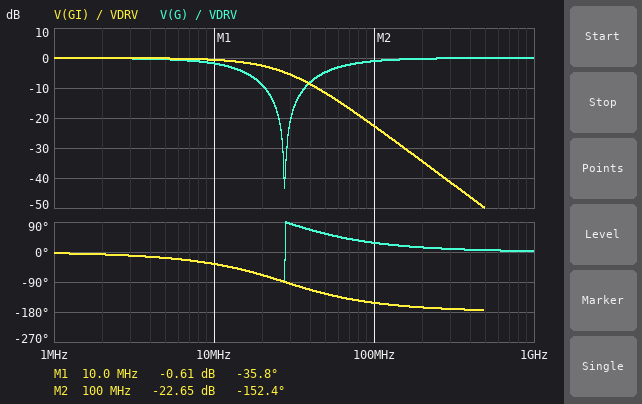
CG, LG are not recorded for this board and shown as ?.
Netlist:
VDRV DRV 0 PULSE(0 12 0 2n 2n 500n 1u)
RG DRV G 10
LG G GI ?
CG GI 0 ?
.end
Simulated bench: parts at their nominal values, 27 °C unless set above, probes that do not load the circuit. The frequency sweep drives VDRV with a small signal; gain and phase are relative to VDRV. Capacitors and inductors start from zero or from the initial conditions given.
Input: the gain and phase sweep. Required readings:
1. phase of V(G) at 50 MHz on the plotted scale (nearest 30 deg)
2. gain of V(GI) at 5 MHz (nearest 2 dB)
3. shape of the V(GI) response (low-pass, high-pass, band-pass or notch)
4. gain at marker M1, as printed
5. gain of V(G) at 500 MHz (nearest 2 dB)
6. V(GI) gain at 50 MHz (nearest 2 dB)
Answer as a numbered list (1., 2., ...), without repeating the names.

1. 60 deg
2. 0 dB
3. low-pass
4. -0.61 dB
5. 0 dB
6. -12 dB
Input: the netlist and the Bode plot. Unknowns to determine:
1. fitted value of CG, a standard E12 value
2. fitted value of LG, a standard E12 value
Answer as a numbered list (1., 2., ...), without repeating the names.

1. 1 nF
2. 33 nH
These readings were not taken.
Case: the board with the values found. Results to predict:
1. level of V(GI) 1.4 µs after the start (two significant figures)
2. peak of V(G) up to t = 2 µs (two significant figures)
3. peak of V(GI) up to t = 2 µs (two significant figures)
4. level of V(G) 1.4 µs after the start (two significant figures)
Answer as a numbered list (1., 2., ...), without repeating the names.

1. 12 V
2. 12 V
3. 12 V
4. 12 V
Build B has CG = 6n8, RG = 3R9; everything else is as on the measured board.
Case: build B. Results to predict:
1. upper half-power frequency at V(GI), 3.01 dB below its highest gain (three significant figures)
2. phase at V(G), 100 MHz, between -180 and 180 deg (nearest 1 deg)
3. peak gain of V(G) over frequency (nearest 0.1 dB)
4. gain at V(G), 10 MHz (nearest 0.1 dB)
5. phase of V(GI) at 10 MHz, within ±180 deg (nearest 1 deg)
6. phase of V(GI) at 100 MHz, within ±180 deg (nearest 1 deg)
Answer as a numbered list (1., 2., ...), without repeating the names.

1. 8.11 MHz
2. 11 deg
3. 0 dB
4. -23.3 dB
5. -86 deg
6. -169 deg
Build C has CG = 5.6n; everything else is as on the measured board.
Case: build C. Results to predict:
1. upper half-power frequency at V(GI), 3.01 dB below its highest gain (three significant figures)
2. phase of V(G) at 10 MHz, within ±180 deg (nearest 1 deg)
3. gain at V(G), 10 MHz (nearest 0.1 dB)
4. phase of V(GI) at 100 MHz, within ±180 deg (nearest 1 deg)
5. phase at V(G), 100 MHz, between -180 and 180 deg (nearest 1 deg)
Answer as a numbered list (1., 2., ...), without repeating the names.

1. 3.02 MHz
2. -86 deg
3. -22.3 dB
4. -154 deg
5. 26 deg
